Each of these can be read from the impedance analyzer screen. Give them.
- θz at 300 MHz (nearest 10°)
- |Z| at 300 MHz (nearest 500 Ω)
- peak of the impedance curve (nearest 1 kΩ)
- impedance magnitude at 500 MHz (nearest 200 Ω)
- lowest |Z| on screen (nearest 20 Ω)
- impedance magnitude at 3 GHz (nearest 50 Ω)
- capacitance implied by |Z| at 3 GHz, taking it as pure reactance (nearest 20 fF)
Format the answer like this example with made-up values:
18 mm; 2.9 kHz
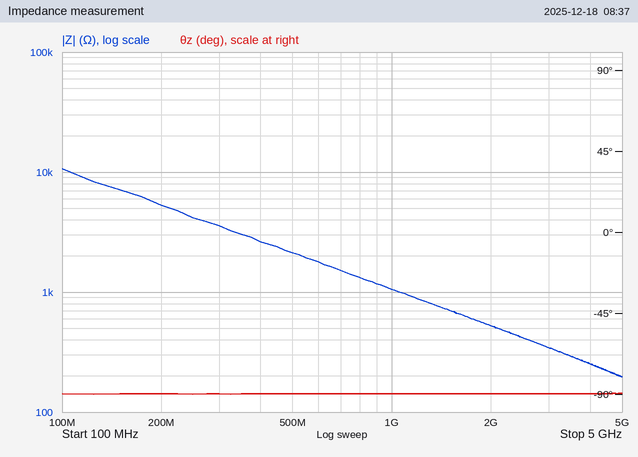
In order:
-90°; 3.5 kΩ; 11 kΩ; 2.2 kΩ; 200 Ω; 350 Ω; 160 fF
